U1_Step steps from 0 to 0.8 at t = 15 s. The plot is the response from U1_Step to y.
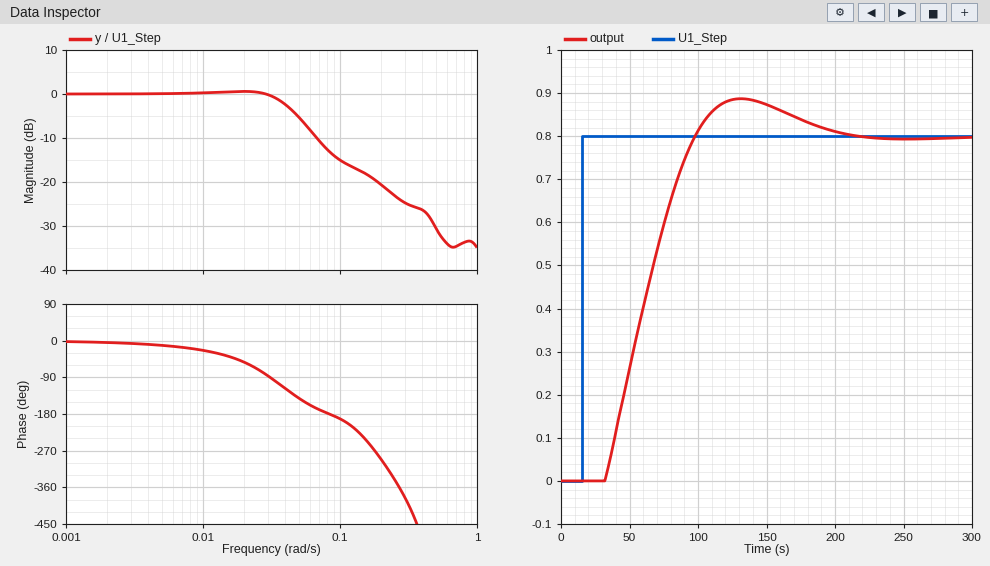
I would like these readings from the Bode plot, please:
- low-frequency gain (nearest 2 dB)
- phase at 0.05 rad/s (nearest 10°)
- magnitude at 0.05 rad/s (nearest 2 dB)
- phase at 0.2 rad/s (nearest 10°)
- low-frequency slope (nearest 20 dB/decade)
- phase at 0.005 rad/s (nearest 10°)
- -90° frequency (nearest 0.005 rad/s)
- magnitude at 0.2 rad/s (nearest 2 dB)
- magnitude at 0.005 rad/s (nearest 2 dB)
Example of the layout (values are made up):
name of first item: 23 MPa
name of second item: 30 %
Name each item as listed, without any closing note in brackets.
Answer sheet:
low-frequency gain: 0 dB
phase at 0.05 rad/s: -140°
magnitude at 0.05 rad/s: -6 dB
phase at 0.2 rad/s: -290°
low-frequency slope: 0 dB/decade
phase at 0.005 rad/s: -10°
-90° frequency: 0.030 rad/s
magnitude at 0.2 rad/s: -20 dB
magnitude at 0.005 rad/s: 0 dB
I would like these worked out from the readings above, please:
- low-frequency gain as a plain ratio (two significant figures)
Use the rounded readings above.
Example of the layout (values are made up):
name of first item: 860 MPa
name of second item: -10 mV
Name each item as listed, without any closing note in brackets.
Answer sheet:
low-frequency gain as a plain ratio: 1.0
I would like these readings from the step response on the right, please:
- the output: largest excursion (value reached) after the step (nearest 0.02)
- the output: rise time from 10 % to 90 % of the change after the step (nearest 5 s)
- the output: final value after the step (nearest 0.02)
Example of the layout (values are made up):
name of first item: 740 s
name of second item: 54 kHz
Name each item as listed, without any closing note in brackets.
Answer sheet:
the output: largest excursion (value reached) after the step: 0.88
the output: rise time from 10 % to 90 % of the change after the step: 50 s
the output: final value after the step: 0.80
